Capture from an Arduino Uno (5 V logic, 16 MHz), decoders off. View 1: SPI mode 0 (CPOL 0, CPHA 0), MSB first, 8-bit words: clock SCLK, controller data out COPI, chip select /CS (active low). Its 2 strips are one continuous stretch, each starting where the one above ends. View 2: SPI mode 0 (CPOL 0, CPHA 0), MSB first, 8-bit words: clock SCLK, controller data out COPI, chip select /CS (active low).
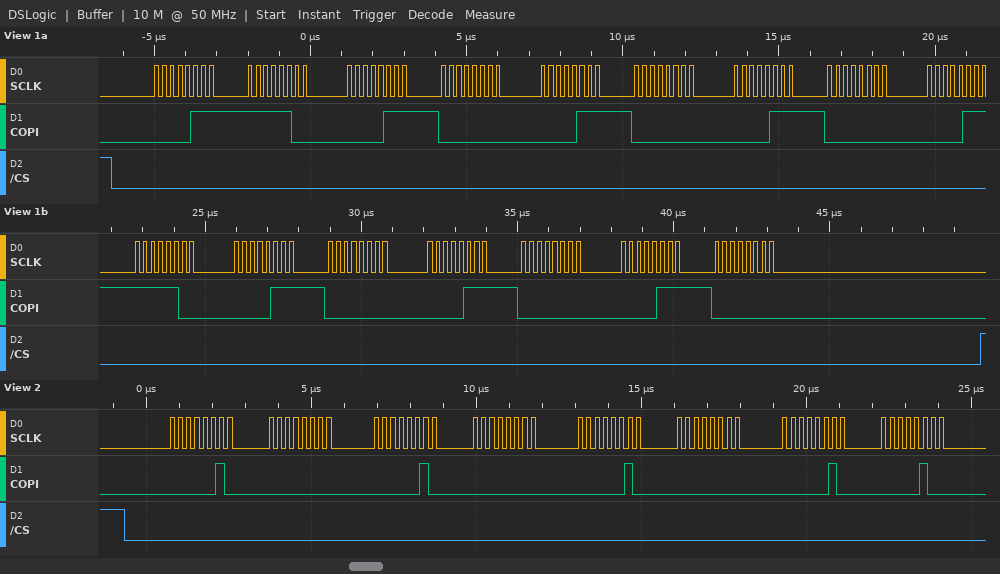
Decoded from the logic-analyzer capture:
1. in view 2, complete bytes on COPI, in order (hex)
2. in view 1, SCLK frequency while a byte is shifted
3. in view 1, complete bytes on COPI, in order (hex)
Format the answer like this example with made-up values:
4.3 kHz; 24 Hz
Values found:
02 00 02 00 02 00 02 04; 4 MHz; 07 FC 07 00 07 00 07 00 07 FC 07 00 07 00 07 00
